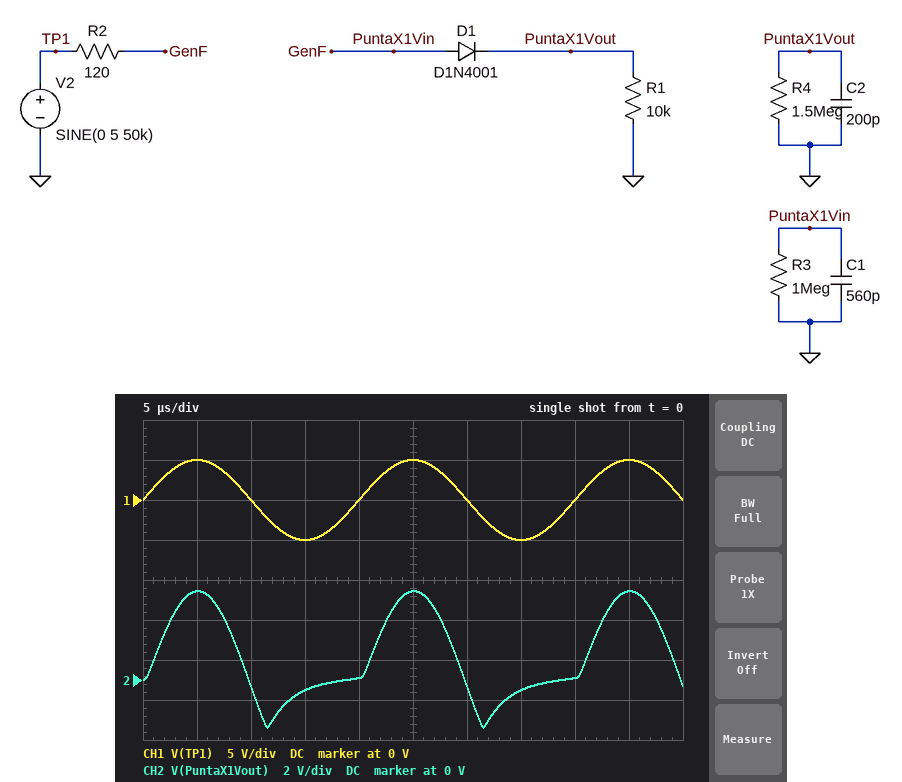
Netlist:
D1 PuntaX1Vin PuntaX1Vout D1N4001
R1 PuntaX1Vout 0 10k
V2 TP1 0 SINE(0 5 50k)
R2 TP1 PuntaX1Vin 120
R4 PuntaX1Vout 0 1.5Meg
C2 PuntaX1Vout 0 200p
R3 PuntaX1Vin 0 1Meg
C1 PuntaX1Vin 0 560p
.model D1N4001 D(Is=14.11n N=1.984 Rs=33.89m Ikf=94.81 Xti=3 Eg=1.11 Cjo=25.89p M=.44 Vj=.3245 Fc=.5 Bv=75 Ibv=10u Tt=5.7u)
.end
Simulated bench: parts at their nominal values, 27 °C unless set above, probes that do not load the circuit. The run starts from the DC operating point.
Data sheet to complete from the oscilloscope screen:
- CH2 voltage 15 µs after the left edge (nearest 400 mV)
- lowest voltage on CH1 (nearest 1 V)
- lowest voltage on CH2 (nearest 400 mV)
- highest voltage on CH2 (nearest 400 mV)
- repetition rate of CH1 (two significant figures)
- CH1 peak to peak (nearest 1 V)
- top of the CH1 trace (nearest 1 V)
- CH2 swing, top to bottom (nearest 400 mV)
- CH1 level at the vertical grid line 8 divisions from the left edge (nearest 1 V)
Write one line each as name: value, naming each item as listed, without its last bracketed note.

CH2 voltage 15 µs after the left edge: -400 mV
lowest voltage on CH1: -5 V
lowest voltage on CH2: -2.4 V
highest voltage on CH2: 4.4 V
repetition rate of CH1: 50 kHz
CH1 peak to peak: 10 V
top of the CH1 trace: 5 V
CH2 swing, top to bottom: 6.8 V
CH1 level at the vertical grid line 8 divisions from the left edge: 0 V
